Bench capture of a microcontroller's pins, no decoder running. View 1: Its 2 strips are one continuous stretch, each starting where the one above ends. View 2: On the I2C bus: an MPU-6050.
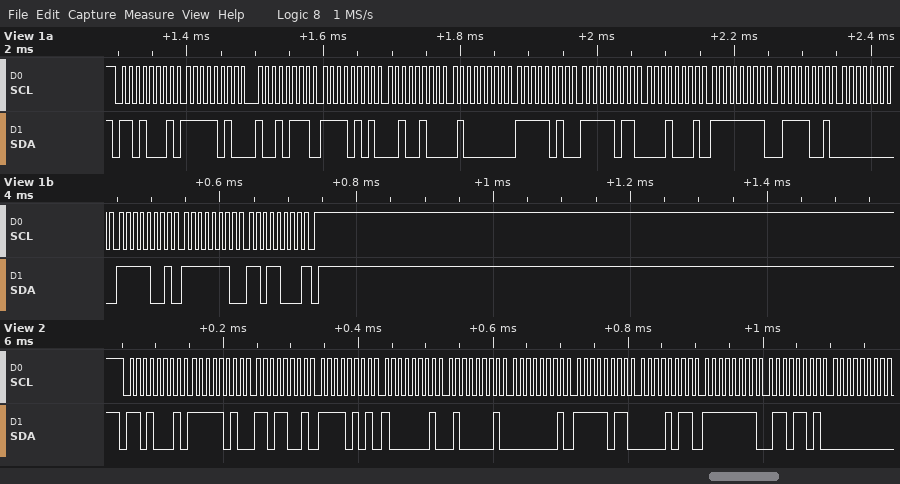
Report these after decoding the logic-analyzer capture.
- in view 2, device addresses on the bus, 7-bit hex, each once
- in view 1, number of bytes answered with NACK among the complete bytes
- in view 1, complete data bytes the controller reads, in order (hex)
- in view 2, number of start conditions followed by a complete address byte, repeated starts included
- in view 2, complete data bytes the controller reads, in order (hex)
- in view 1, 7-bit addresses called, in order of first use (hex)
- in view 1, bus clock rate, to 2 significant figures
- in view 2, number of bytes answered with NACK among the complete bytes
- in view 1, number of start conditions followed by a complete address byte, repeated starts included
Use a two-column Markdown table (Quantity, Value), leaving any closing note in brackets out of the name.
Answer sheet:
| Quantity | Value |
|---|---|
| in view 2, device addresses on the bus, 7-bit hex, each once | 0x68 |
| in view 1, number of bytes answered with NACK among the complete bytes | 1 |
| in view 1, complete data bytes the controller reads, in order | FA 97 F5 24 40 FA FB 11 FF 79 00 F9 FE D8 |
| in view 2, number of start conditions followed by a complete address byte, repeated starts included | 1 |
| in view 2, complete data bytes the controller reads, in order | FA D9 F5 81 41 01 FB 0B FF 6D 00 |
| in view 1, 7-bit addresses called, in order of first use | 0x68 |
| in view 1, bus clock rate, to 2 significant figures | 100 kHz |
| in view 2, number of bytes answered with NACK among the complete bytes | 0 |
| in view 1, number of start conditions followed by a complete address byte, repeated starts included | 1 |
